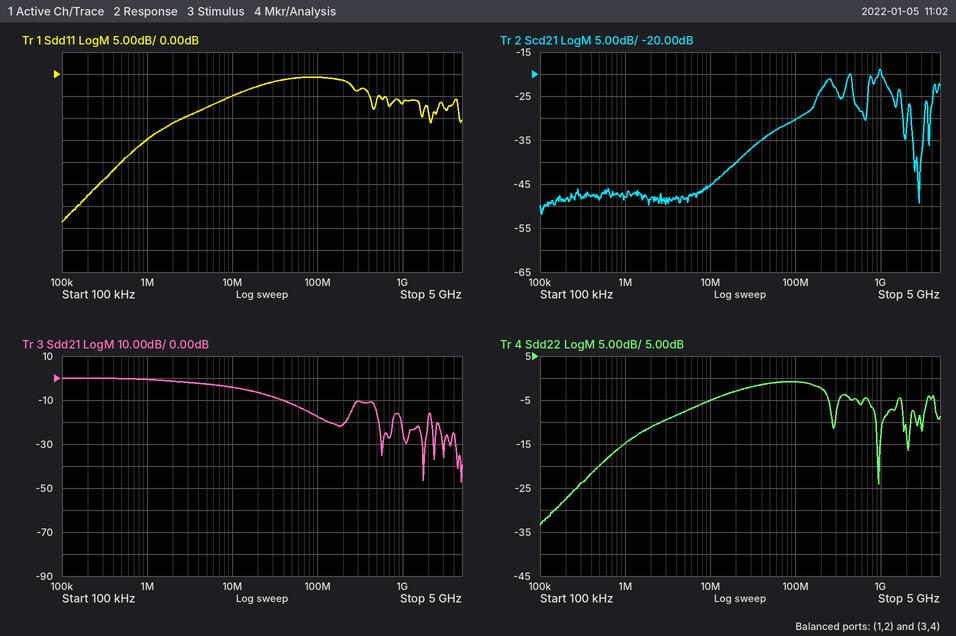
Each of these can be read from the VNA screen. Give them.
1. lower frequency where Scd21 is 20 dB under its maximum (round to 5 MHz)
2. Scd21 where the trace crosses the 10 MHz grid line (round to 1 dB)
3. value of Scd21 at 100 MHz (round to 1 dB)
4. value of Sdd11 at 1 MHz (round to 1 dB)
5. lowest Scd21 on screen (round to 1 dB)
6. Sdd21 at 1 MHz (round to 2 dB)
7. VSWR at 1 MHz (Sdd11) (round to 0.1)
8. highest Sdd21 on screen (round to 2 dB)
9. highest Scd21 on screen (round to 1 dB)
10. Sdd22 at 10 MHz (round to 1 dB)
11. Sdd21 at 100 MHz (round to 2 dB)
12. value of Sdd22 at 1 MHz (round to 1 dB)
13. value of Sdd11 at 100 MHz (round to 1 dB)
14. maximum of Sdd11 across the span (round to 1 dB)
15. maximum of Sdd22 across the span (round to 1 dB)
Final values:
25 MHz
-45 dB
-30 dB
-15 dB
-52 dB
0 dB
1.4
0 dB
-19 dB
-5 dB
-18 dB
-15 dB
-1 dB
-1 dB
-1 dB
